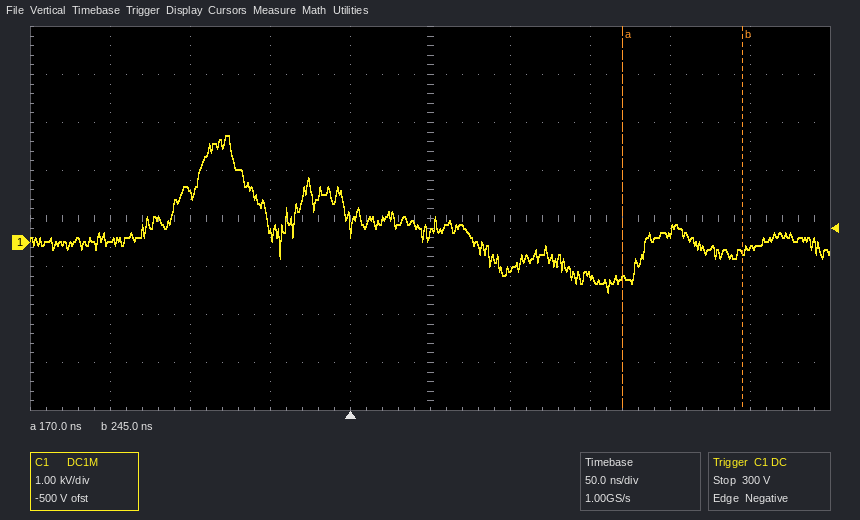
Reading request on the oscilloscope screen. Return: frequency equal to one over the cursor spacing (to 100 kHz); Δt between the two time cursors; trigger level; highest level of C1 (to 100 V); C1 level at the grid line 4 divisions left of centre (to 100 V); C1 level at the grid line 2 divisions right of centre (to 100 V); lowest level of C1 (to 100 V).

13.3 MHz
75 ns
300 V
2.2 kV
0.0 kV
-700 V
-1.0 kV
